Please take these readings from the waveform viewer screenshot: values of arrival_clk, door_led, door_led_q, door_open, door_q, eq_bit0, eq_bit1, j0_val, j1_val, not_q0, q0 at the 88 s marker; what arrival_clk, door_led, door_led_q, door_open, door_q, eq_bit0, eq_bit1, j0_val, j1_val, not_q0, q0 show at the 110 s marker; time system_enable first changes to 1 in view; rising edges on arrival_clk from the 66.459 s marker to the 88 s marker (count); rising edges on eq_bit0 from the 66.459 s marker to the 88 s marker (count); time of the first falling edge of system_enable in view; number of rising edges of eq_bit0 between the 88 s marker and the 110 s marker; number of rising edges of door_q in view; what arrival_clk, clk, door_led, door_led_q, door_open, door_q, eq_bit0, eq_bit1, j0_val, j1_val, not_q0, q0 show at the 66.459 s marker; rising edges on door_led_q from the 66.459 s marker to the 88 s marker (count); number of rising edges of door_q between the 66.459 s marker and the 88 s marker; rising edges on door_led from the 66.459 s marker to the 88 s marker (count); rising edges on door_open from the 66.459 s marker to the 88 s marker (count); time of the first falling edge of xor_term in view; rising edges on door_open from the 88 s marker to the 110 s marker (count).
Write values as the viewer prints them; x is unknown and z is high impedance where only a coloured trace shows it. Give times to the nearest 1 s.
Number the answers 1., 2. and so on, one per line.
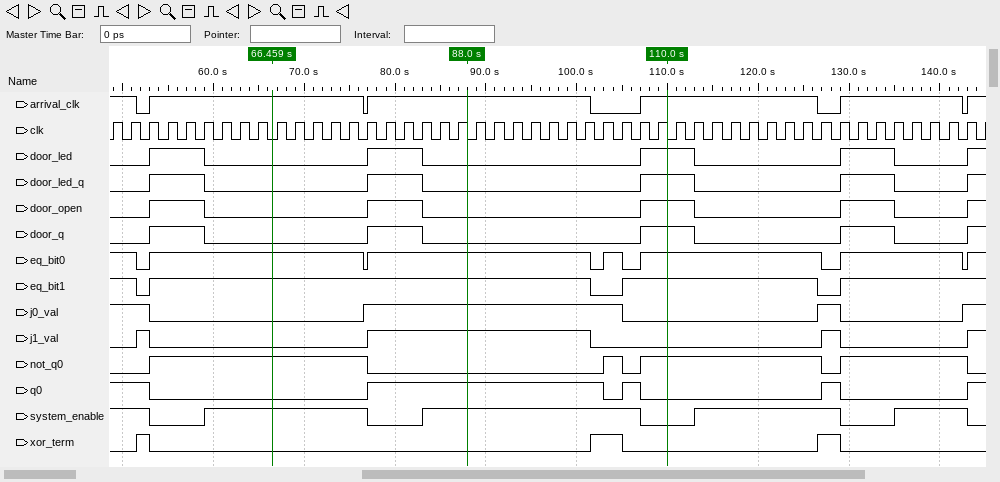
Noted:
1. arrival_clk=1, door_led=0, door_led_q=0, door_open=0, door_q=0, eq_bit0=1, eq_bit1=1, j0_val=1, j1_val=1, not_q0=0, q0=1
2. arrival_clk=1, door_led=1, door_led_q=1, door_open=1, door_q=1, eq_bit0=1, eq_bit1=1, j0_val=0, j1_val=0, not_q0=1, q0=0
3. 59 s
4. 1
5. 1
6. 53 s
7. 2
8. 5
9. arrival_clk=1, clk=0, door_led=0, door_led_q=0, door_open=0, door_q=0, eq_bit0=1, eq_bit1=1, j0_val=0, j1_val=0, not_q0=1, q0=0
10. 1
11. 1
12. 1
13. 1
14. 53 s
15. 1
